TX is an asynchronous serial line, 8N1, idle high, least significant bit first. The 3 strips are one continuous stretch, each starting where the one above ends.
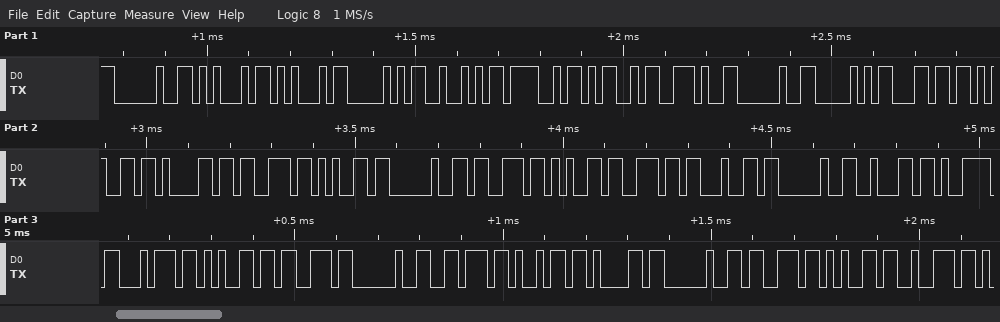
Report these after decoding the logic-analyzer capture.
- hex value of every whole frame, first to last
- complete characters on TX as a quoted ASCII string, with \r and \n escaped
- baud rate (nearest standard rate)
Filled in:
20 45 45 50 52 4F 4D 2E 20 50 6C 65 61 73 65 20 73 65 6E 64 20 62 79 74 65 73 20 76 69 61 20 73 65 72
" EEPROM. Please send bytes via ser"
57600 baud
